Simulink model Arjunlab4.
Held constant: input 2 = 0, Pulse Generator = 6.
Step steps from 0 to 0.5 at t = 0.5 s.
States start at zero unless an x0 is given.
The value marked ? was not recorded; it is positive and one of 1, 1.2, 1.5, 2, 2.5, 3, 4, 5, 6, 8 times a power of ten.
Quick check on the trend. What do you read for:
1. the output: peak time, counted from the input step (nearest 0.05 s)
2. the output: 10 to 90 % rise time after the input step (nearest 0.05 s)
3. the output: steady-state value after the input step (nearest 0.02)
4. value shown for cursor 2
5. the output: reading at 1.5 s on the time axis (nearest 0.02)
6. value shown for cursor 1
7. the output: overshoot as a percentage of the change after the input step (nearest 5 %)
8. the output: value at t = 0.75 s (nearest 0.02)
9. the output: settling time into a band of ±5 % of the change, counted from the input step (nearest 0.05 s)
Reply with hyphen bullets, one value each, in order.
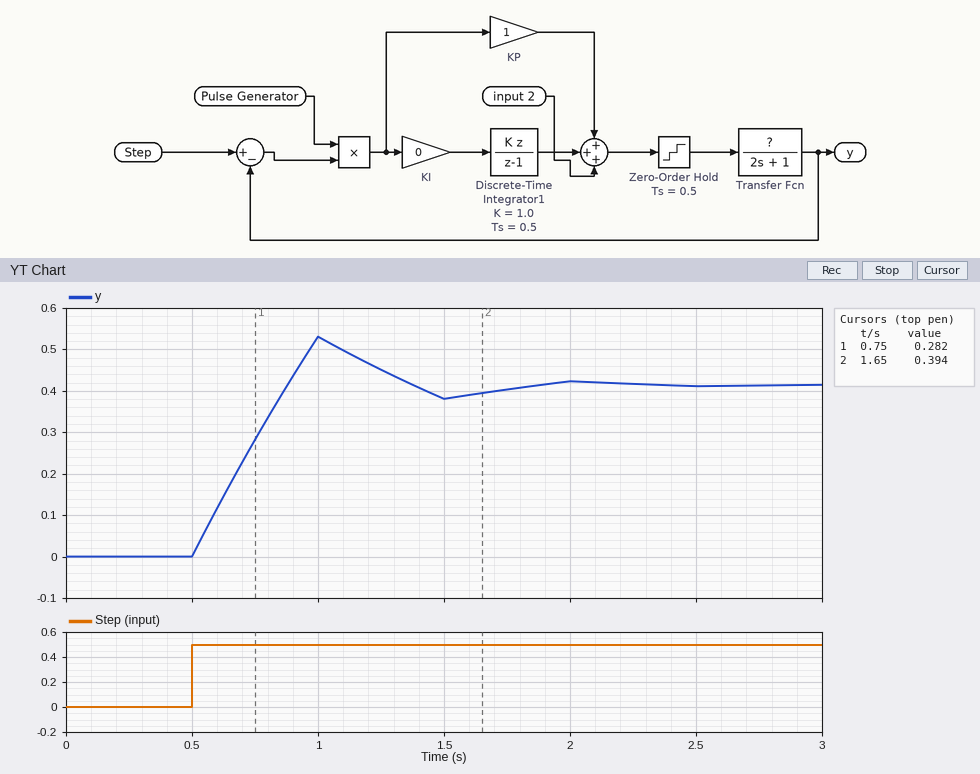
- 0.50 s
- 0.30 s
- 0.42
- 0.394
- 0.38
- 0.282
- 30 %
- 0.28
- 1.15 s
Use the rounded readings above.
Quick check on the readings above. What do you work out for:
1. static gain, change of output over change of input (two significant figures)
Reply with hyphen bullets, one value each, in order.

- 0.84
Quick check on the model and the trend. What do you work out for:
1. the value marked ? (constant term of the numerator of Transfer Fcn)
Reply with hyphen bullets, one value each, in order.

- 0.8
